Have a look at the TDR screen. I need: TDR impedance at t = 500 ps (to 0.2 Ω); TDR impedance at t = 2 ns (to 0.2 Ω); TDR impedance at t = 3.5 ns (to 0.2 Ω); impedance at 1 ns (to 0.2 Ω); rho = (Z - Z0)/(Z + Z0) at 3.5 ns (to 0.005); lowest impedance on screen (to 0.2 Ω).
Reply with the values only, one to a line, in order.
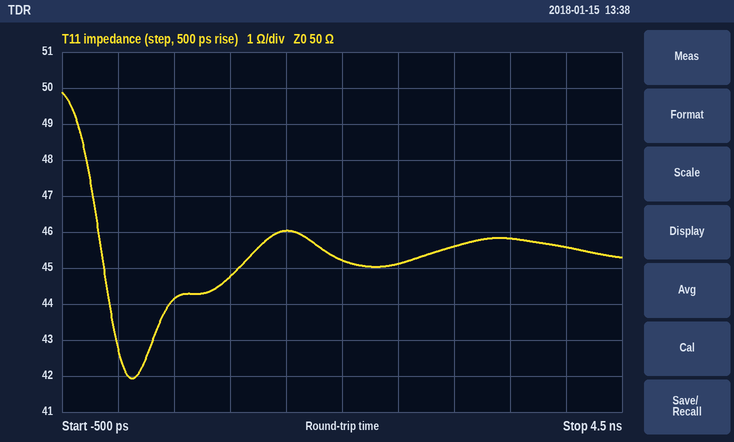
44.2 Ω
45.2 Ω
45.8 Ω
44.8 Ω
-0.045
42.0 Ω
